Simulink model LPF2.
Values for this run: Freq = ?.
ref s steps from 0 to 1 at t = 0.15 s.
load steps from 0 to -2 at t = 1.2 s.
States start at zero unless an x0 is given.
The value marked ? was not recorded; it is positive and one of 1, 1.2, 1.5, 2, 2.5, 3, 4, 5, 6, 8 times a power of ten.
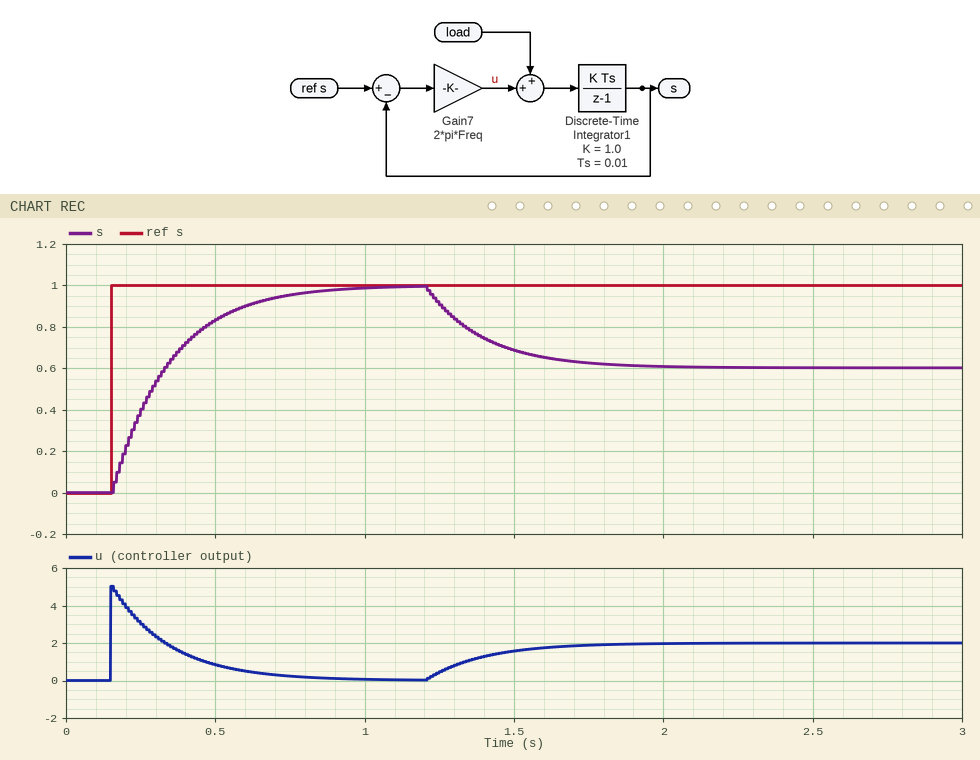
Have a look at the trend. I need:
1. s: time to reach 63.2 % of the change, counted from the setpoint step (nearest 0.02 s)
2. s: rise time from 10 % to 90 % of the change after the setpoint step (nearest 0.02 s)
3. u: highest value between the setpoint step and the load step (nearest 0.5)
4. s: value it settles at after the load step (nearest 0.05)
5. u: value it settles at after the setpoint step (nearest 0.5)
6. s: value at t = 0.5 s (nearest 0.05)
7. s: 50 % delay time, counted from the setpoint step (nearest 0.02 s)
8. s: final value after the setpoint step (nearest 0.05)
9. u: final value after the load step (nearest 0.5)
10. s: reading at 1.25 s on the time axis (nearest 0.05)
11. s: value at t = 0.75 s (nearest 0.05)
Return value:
0.20 s
0.42 s
5.0
0.60
0.0
0.85
0.14 s
1.00
2.0
0.90
0.95
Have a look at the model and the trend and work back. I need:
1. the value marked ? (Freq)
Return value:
0.8
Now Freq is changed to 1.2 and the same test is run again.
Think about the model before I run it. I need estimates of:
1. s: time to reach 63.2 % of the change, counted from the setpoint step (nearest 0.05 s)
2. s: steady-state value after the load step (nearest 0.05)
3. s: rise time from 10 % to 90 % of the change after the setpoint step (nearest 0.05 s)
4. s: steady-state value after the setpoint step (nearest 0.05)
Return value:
0.15 s
0.75
0.30 s
1.00
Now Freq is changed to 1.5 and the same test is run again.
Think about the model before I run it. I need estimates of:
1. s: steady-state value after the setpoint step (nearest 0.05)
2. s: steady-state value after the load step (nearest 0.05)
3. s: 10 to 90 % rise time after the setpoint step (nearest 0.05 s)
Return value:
1.00
0.80
0.20 s
